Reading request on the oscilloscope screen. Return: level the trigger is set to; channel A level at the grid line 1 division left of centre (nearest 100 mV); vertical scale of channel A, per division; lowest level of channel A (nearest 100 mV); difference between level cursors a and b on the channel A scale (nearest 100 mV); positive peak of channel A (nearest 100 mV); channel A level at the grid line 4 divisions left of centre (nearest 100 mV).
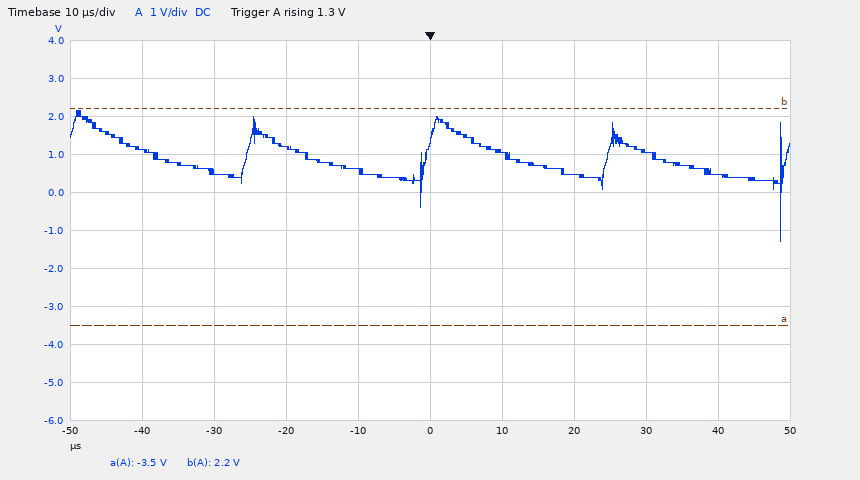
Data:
1.3 V
600 mV
1 V
-1.3 V
5.7 V
2.2 V
1.1 V
